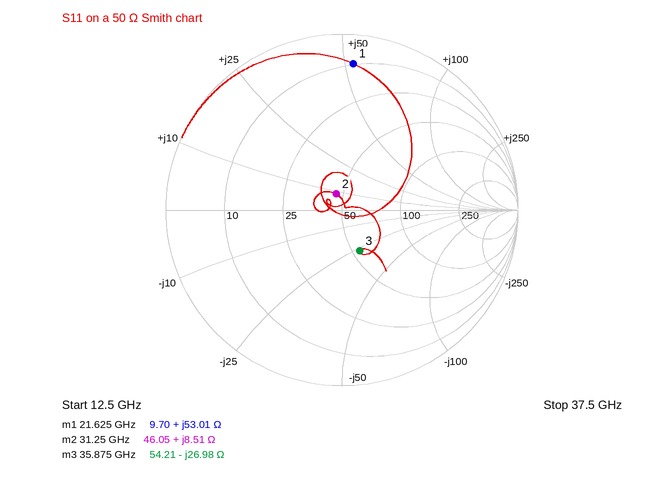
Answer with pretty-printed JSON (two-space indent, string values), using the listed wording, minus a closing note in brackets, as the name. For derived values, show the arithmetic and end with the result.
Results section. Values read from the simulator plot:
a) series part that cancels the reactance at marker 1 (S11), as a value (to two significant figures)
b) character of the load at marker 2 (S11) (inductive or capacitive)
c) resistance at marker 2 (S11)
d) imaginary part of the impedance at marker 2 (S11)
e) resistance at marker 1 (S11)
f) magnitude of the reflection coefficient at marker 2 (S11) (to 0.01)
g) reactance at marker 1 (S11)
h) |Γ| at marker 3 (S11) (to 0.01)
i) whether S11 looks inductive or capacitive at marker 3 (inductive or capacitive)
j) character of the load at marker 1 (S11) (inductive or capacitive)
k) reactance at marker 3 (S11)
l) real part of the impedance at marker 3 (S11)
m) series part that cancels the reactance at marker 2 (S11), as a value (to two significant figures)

{
  "series part that cancels the reactance at marker 1 (S11), as a value": "C = 1/(2π × 21.625 GHz × 53.01 Ω) ≈ 139 fF, so 140 fF to two significant figures",
  "character of the load at marker 2 (S11)": "inductive",
  "resistance at marker 2": "46.05 Ω",
  "imaginary part of the impedance at marker 2": "+8.51 Ω",
  "resistance at marker 1": "9.70 Ω",
  "magnitude of the reflection coefficient at marker 2 (S11)": "0.10",
  "reactance at marker 1": "+53.01 Ω",
  "|Γ| at marker 3 (S11)": "0.25",
  "whether S11 looks inductive or capacitive at marker 3": "capacitive",
  "character of the load at marker 1 (S11)": "inductive",
  "reactance at marker 3": "-26.98 Ω",
  "real part of the impedance at marker 3": "54.21 Ω",
  "series part that cancels the reactance at marker 2 (S11), as a value": "C = 1/(2π × 31.25 GHz × 8.51 Ω) ≈ 598 fF, so 600 fF to two significant figures"
}
